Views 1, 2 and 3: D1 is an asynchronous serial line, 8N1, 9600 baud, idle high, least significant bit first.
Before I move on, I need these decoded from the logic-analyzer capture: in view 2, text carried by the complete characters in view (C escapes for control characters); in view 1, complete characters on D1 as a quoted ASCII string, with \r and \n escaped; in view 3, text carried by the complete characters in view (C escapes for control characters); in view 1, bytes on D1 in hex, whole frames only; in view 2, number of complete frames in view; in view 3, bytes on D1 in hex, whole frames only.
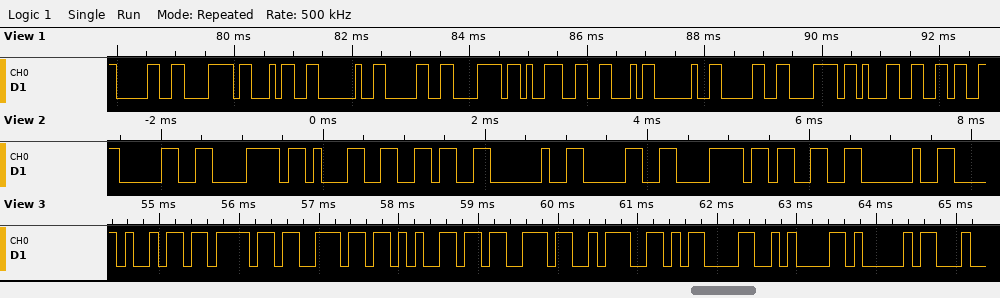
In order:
"0x16 0x3 "
"0x4 0x9F 0x16"
"iones:\r\nA"
0x30 0x78 0x34 0x20 0x30 0x78 0x39 0x46 0x20 0x30 0x78 0x31 0x36
9
0x69 0x6F 0x6E 0x65 0x73 0x3A 0x0D 0x0A 0x41
